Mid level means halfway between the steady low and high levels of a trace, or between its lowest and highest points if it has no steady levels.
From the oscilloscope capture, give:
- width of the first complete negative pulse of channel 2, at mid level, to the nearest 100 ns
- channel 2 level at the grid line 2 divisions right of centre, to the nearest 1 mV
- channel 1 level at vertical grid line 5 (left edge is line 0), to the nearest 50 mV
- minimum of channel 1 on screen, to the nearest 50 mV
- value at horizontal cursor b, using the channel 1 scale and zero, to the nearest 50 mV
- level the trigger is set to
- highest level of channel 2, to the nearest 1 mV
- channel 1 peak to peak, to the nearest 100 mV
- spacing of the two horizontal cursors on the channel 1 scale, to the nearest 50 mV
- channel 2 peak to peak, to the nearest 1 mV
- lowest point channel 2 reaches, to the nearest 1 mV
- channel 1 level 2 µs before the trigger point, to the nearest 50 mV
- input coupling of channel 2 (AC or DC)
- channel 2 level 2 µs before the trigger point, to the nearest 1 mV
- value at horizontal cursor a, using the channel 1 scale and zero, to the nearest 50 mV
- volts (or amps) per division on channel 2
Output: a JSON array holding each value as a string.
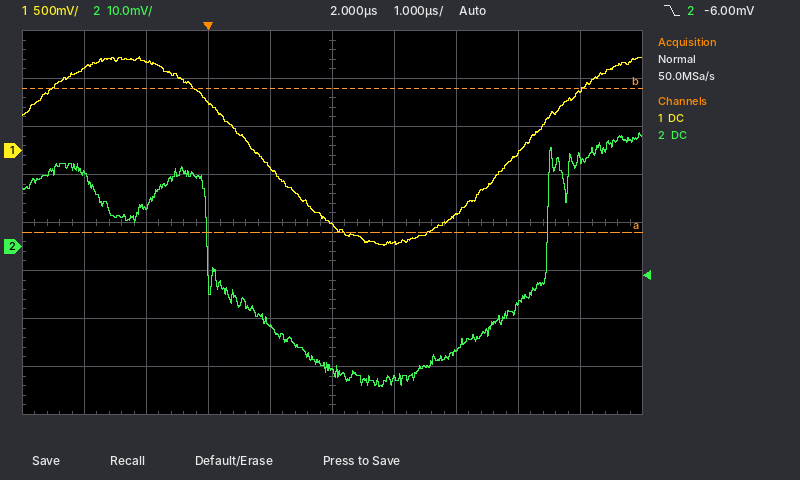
["5.5 µs", "-22 mV", "-750 mV", "-1.00 V", "650 mV", "-6.00 mV", "24 mV", "2.00 V", "1.50 V", "53 mV", "-29 mV", "850 mV", "DC", "15 mV", "-850 mV", "10 mV"]
